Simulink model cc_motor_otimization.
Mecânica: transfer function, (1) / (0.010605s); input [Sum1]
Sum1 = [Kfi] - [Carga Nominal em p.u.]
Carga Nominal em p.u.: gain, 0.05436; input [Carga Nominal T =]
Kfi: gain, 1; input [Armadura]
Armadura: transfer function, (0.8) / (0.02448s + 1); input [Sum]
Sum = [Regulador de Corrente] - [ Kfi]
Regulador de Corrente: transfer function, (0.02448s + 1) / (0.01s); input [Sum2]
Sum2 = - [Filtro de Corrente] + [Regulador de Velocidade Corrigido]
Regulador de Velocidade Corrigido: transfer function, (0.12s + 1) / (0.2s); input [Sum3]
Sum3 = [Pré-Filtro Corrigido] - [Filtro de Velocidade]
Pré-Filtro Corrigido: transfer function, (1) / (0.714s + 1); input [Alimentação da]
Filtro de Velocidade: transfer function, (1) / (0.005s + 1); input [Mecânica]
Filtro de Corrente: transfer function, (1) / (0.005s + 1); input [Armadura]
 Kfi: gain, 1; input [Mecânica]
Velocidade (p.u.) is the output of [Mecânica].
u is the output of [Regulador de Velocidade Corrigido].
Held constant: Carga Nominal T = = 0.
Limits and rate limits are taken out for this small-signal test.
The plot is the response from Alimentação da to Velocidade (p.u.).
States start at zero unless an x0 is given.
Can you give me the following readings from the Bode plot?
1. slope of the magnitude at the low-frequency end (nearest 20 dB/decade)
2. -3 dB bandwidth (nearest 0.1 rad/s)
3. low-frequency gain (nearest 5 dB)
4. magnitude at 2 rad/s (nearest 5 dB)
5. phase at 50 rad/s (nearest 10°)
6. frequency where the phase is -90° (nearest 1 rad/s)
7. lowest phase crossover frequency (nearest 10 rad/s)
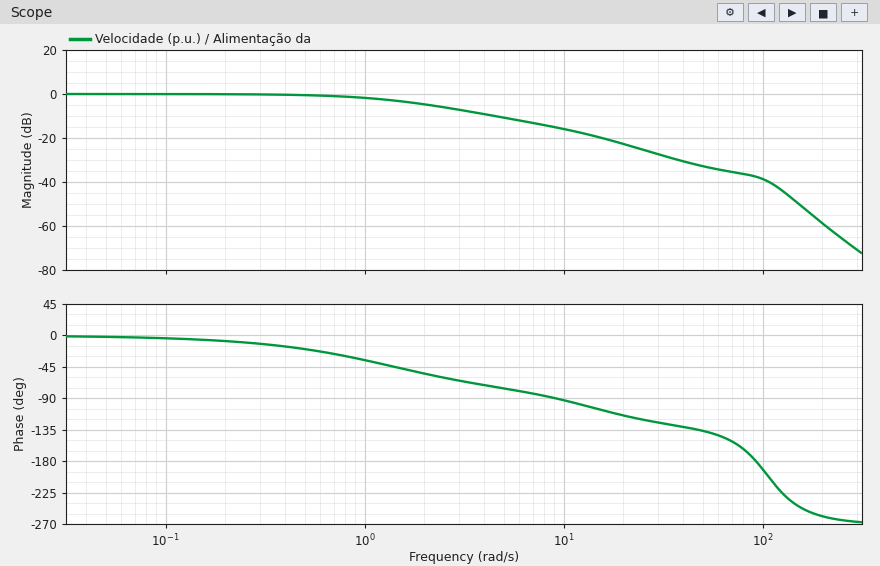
0 dB/decade
1.4 rad/s
0 dB
-5 dB
-140°
9 rad/s
90 rad/s
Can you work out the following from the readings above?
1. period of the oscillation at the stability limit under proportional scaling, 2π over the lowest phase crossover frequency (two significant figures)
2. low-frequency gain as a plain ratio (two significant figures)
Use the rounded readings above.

0.070 s
1.0
